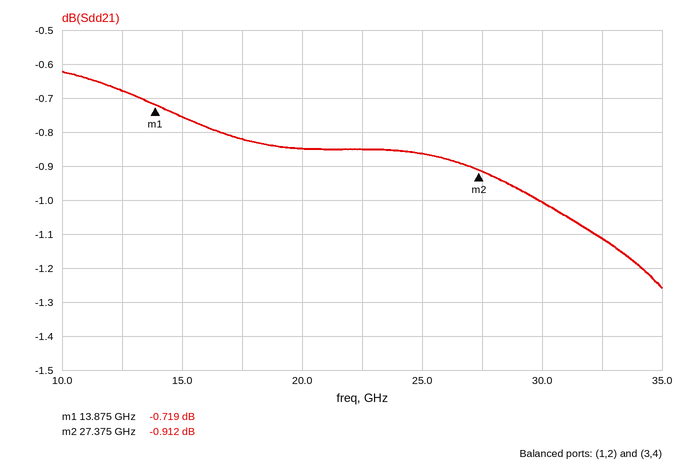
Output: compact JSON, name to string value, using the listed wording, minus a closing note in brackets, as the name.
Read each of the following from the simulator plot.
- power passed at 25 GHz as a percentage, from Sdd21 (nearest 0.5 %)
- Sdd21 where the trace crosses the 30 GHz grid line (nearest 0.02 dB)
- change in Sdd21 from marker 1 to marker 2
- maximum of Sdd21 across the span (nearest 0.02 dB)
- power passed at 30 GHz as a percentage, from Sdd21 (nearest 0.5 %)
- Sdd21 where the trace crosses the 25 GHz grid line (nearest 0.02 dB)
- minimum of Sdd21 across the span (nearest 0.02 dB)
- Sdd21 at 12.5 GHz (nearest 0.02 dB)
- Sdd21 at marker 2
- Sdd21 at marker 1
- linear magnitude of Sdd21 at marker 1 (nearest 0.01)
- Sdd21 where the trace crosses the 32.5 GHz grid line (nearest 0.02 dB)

{"power passed at 25 GHz as a percentage, from Sdd21": "82.0 %", "Sdd21 where the trace crosses the 30 GHz grid line": "-1.00 dB", "change in Sdd21 from marker 1 to marker 2": "-0.193 dB", "maximum of Sdd21 across the span": "-0.62 dB", "power passed at 30 GHz as a percentage, from Sdd21": "79.5 %", "Sdd21 where the trace crosses the 25 GHz grid line": "-0.86 dB", "minimum of Sdd21 across the span": "-1.26 dB", "Sdd21 at 12.5 GHz": "-0.68 dB", "Sdd21 at marker 2": "-0.912 dB", "Sdd21 at marker 1": "-0.719 dB", "linear magnitude of Sdd21 at marker 1": "0.92", "Sdd21 where the trace crosses the 32.5 GHz grid line": "-1.12 dB"}
